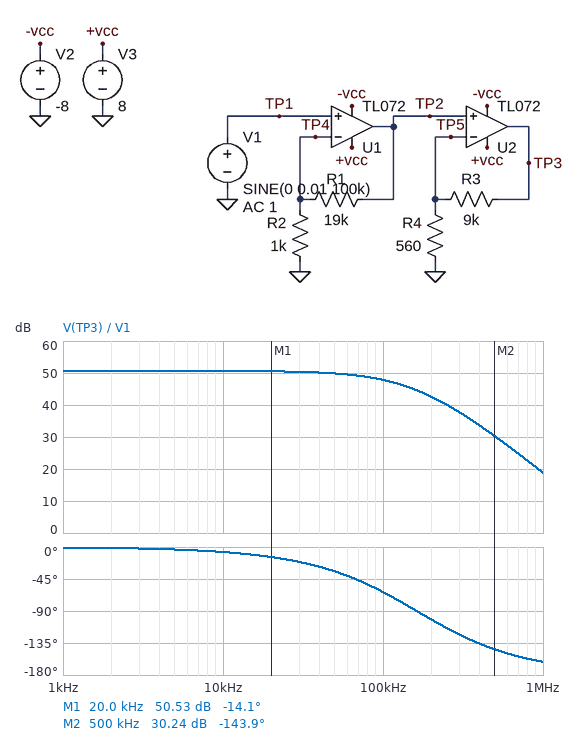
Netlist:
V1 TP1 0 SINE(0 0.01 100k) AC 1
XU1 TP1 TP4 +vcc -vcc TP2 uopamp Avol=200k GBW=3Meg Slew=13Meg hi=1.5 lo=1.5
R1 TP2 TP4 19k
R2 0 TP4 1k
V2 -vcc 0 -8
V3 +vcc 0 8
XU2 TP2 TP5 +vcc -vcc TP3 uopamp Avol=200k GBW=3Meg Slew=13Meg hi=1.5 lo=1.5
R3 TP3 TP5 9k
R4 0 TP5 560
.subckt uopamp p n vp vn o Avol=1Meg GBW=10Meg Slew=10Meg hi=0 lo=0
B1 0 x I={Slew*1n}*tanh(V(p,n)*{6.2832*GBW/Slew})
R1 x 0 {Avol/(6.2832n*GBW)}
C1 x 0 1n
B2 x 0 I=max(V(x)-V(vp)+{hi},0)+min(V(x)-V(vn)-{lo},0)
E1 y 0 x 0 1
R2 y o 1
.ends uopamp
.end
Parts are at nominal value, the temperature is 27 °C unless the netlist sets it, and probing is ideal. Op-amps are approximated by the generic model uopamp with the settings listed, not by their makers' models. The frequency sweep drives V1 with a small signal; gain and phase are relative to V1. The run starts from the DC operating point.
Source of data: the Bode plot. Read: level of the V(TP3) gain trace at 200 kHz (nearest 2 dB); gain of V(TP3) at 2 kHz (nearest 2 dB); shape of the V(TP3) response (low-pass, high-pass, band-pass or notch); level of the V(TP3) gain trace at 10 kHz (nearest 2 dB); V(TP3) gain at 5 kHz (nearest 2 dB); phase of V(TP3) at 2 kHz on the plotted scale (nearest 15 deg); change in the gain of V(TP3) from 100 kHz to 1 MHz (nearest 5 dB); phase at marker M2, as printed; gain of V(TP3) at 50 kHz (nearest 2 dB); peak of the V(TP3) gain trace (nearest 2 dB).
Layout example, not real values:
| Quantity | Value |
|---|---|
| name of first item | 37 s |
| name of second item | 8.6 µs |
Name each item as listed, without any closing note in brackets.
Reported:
| Quantity | Value |
|---|---|
| level of the V(TP3) gain trace at 200 kHz | 42 dB |
| gain of V(TP3) at 2 kHz | 50 dB |
| shape of the V(TP3) response | low-pass |
| level of the V(TP3) gain trace at 10 kHz | 50 dB |
| V(TP3) gain at 5 kHz | 50 dB |
| phase of V(TP3) at 2 kHz on the plotted scale | 0 deg |
| change in the gain of V(TP3) from 100 kHz to 1 MHz | -30 dB |
| phase at marker M2, as printed | -143.9 deg |
| gain of V(TP3) at 50 kHz | 50 dB |
| peak of the V(TP3) gain trace | 50 dB |
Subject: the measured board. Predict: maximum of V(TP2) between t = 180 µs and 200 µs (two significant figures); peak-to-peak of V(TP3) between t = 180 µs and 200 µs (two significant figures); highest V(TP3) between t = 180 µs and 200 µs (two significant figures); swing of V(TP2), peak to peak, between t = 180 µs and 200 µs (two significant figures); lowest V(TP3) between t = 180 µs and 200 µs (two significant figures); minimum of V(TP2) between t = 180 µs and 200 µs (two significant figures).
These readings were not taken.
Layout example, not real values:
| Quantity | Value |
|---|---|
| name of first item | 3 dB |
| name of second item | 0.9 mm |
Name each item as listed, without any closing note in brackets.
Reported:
| Quantity | Value |
|---|---|
| maximum of V(TP2) between t = 180 µs and 200 µs | 170 mV |
| peak-to-peak of V(TP3) between t = 180 µs and 200 µs | 4.9 V |
| highest V(TP3) between t = 180 µs and 200 µs | 2.5 V |
| swing of V(TP2), peak to peak, between t = 180 µs and 200 µs | 330 mV |
| lowest V(TP3) between t = 180 µs and 200 µs | -2.5 V |
| minimum of V(TP2) between t = 180 µs and 200 µs | -170 mV |
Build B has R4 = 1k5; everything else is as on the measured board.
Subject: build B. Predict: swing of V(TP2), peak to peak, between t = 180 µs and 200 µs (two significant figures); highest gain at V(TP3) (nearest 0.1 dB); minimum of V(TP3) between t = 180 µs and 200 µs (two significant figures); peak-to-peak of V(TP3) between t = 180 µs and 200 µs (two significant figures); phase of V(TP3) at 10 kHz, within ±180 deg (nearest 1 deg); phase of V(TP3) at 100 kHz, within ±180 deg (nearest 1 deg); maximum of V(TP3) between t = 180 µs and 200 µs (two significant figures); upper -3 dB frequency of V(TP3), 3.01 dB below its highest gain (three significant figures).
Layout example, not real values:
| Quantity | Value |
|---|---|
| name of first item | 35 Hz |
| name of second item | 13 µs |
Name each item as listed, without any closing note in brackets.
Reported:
| Quantity | Value |
|---|---|
| swing of V(TP2), peak to peak, between t = 180 µs and 200 µs | 330 mV |
| highest gain at V(TP3) | 42.9 dB |
| minimum of V(TP3) between t = 180 µs and 200 µs | -1.1 V |
| peak-to-peak of V(TP3) between t = 180 µs and 200 µs | 2.3 V |
| phase of V(TP3) at 10 kHz, within ±180 deg | -5 deg |
| phase of V(TP3) at 100 kHz, within ±180 deg | -47 deg |
| maximum of V(TP3) between t = 180 µs and 200 µs | 1.1 V |
| upper -3 dB frequency of V(TP3), 3.01 dB below its highest gain | 136 kHz |
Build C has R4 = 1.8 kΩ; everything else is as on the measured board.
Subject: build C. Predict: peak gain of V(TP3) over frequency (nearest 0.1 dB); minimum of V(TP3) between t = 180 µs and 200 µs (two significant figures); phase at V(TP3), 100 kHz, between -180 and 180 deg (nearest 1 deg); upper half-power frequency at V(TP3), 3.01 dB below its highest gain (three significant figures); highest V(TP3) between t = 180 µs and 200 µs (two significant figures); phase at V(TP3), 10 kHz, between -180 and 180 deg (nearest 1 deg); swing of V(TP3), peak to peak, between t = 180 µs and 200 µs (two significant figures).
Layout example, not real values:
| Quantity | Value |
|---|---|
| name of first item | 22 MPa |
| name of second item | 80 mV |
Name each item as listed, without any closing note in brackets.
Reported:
| Quantity | Value |
|---|---|
| peak gain of V(TP3) over frequency | 41.6 dB |
| minimum of V(TP3) between t = 180 µs and 200 µs | -980 mV |
| phase at V(TP3), 100 kHz, between -180 and 180 deg | -45 deg |
| upper half-power frequency at V(TP3), 3.01 dB below its highest gain | 139 kHz |
| highest V(TP3) between t = 180 µs and 200 µs | 980 mV |
| phase at V(TP3), 10 kHz, between -180 and 180 deg | -5 deg |
| swing of V(TP3), peak to peak, between t = 180 µs and 200 µs | 2.0 V |
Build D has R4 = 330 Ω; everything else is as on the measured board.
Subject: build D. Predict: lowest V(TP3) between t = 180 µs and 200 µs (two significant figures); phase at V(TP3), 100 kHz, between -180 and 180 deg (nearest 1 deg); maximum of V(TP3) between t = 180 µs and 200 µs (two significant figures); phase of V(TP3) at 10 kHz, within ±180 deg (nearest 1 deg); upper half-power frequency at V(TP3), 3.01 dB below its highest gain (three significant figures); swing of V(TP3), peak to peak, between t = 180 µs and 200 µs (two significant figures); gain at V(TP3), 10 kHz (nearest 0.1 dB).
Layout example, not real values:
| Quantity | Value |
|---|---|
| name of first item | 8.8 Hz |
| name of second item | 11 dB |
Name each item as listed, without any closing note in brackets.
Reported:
| Quantity | Value |
|---|---|
| lowest V(TP3) between t = 180 µs and 200 µs | -3.4 V |
| phase at V(TP3), 100 kHz, between -180 and 180 deg | -77 deg |
| maximum of V(TP3) between t = 180 µs and 200 µs | 3.4 V |
| phase of V(TP3) at 10 kHz, within ±180 deg | -9 deg |
| upper half-power frequency at V(TP3), 3.01 dB below its highest gain | 79.5 kHz |
| swing of V(TP3), peak to peak, between t = 180 µs and 200 µs | 6.8 V |
| gain at V(TP3), 10 kHz | 55.0 dB |
